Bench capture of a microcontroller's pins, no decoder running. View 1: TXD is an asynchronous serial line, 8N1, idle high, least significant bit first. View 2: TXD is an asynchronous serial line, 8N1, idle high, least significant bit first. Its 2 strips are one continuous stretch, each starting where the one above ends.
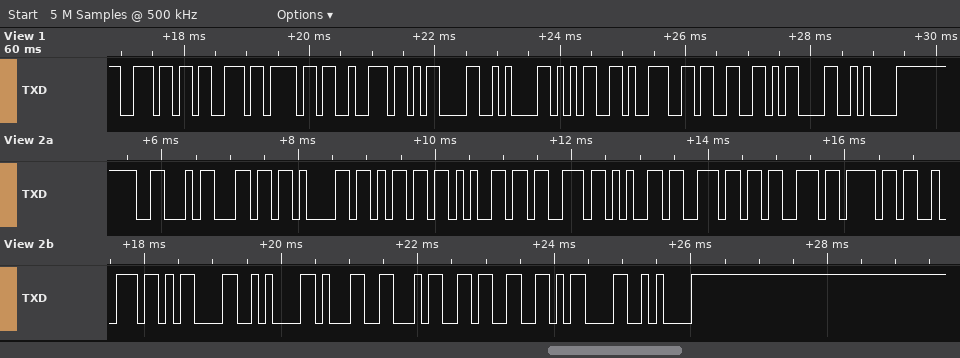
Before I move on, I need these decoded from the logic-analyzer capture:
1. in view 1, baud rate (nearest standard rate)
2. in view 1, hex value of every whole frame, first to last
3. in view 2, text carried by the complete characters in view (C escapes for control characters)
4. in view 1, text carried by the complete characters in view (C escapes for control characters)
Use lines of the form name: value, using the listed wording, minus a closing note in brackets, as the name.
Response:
in view 1, baud rate: 9600 baud
in view 1, hex value of every whole frame, first to last: 6E 73 6F 72 0D 0A 35 39 33 0D 0A
in view 2, text carried by the complete characters in view: "Flamesensor\r\n143\r\n"
in view 1, text carried by the complete characters in view: "nsor\r\n593\r\n"
